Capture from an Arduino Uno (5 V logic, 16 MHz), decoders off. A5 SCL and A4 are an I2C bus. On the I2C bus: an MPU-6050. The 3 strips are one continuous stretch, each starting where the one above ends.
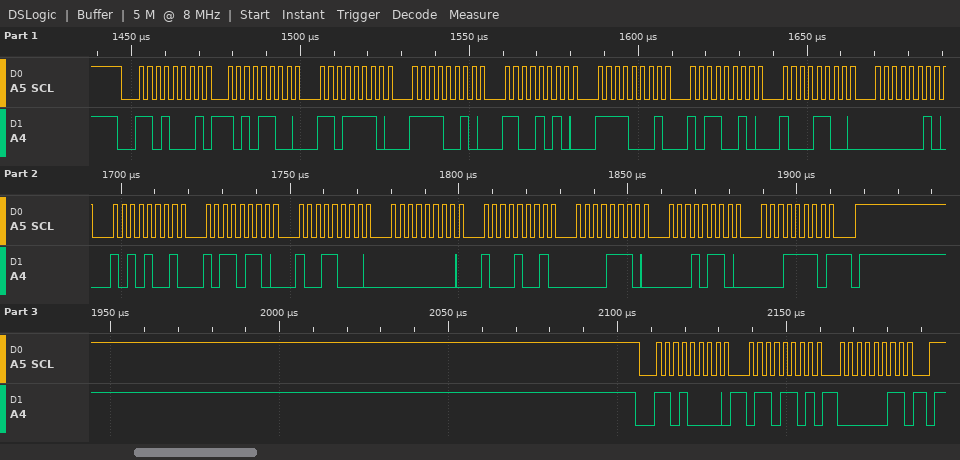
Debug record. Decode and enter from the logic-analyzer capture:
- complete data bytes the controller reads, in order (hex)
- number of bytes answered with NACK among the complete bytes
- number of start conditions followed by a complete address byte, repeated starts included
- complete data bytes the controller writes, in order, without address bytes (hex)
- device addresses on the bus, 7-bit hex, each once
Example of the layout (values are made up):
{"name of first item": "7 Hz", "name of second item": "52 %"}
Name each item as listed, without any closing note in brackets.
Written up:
{"complete data bytes the controller reads, in order": "AC DE F2 CA F1 B2 8C 02 A9 B6 98 00 89 0E 16 1E", "number of bytes answered with NACK among the complete bytes": "1", "number of start conditions followed by a complete address byte, repeated starts included": "2", "complete data bytes the controller writes, in order, without address bytes": "6D 03", "device addresses on the bus, 7-bit hex, each once": "0x68"}
